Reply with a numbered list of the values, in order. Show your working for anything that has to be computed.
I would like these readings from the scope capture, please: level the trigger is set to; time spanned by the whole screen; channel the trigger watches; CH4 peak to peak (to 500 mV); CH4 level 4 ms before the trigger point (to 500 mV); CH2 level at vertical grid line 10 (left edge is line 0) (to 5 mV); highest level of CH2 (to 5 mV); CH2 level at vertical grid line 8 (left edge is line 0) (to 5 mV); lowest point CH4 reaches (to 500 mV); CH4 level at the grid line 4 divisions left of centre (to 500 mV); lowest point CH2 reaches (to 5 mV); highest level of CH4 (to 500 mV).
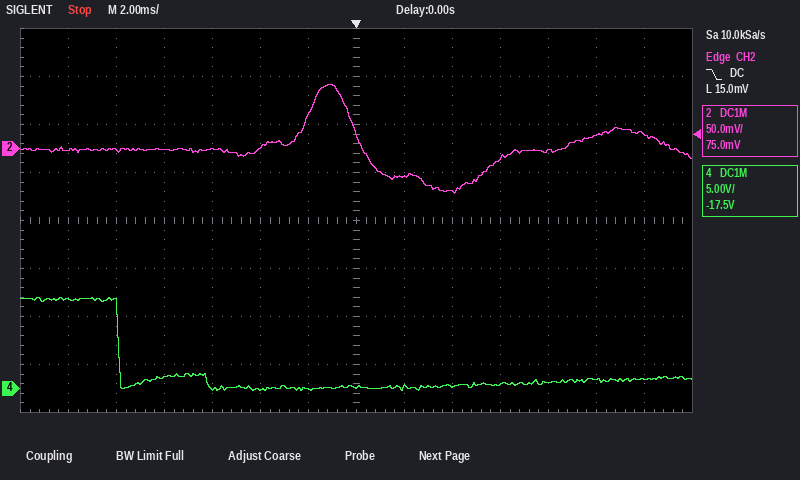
1. 15.0 mV
2. 28 ms
3. CH2
4. 9.5 V − (0.0 V) = 9.5 V
5. 0.0 V
6. -10 mV
7. 65 mV
8. -30 mV
9. 0.0 V
10. 1.0 V
11. -45 mV
12. 9.5 V
